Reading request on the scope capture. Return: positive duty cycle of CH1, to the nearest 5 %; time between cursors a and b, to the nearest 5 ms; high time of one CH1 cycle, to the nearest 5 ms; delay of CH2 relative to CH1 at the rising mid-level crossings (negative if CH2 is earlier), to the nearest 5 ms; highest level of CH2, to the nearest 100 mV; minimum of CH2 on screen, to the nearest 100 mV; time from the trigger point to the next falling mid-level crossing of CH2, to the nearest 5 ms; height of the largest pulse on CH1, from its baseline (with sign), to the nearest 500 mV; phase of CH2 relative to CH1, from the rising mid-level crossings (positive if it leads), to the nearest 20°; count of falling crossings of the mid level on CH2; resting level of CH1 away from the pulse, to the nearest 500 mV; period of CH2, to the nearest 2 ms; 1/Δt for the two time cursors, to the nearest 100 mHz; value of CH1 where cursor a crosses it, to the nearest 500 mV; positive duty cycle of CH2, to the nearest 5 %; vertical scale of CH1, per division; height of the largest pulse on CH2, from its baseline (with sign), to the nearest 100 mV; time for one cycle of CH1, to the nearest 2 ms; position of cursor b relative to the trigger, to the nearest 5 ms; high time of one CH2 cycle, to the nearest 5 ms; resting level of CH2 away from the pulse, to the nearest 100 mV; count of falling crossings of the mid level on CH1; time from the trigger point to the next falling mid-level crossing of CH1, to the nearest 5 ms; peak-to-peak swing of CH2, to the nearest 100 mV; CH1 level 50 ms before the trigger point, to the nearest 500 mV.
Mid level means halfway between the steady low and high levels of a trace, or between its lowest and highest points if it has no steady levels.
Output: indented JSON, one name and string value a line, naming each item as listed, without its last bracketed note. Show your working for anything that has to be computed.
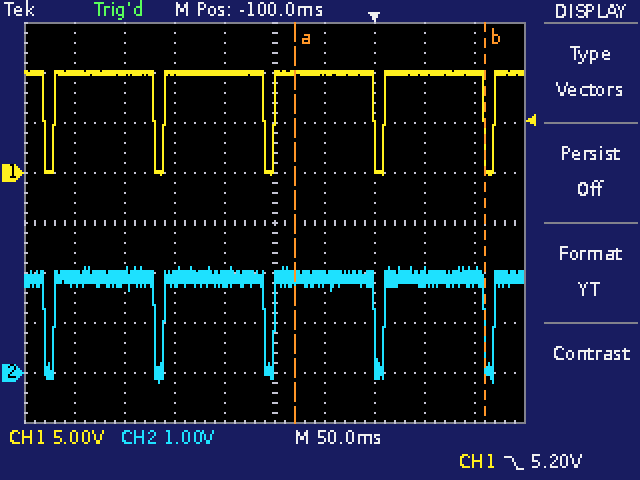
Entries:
{
  "positive duty cycle of CH1, to the nearest 5 %": "100 ms / 110 ms ≈ 90.9 %, so 90 % to the nearest 5 %",
  "time between cursors a and b, to the nearest 5 ms": "190 ms",
  "high time of one CH1 cycle, to the nearest 5 ms": "100 ms",
  "delay of CH2 relative to CH1 at the rising mid-level crossings (negative if CH2 is earlier), to the nearest 5 ms": "0 ms",
  "highest level of CH2, to the nearest 100 mV": "2.1 V",
  "minimum of CH2 on screen, to the nearest 100 mV": "-200 mV",
  "time from the trigger point to the next falling mid-level crossing of CH2, to the nearest 5 ms": "110 ms",
  "height of the largest pulse on CH1, from its baseline (with sign), to the nearest 500 mV": "-10.0 V",
  "phase of CH2 relative to CH1, from the rising mid-level crossings (positive if it leads), to the nearest 20°": "−360° × (0 ms) / 110 ms ≈ 0°",
  "count of falling crossings of the mid level on CH2": "5",
  "resting level of CH1 away from the pulse, to the nearest 500 mV": "10.0 V",
  "period of CH2, to the nearest 2 ms": "110 ms",
  "1/Δt for the two time cursors, to the nearest 100 mHz": "1 / 190 ms ≈ 5.3 Hz",
  "value of CH1 where cursor a crosses it, to the nearest 500 mV": "10.0 V",
  "positive duty cycle of CH2, to the nearest 5 %": "100 ms / 110 ms ≈ 90.9 %, so 90 % to the nearest 5 %",
  "vertical scale of CH1, per division": "5 V",
  "height of the largest pulse on CH2, from its baseline (with sign), to the nearest 100 mV": "-200 mV − (1.9 V) = -2.1 V",
  "time for one cycle of CH1, to the nearest 2 ms": "110 ms",
  "position of cursor b relative to the trigger, to the nearest 5 ms": "+110 ms",
  "high time of one CH2 cycle, to the nearest 5 ms": "100 ms",
  "resting level of CH2 away from the pulse, to the nearest 100 mV": "1.9 V",
  "count of falling crossings of the mid level on CH1": "5",
  "time from the trigger point to the next falling mid-level crossing of CH1, to the nearest 5 ms": "110 ms",
  "peak-to-peak swing of CH2, to the nearest 100 mV": "2.1 V − (-200 mV) = 2.3 V",
  "CH1 level 50 ms before the trigger point, to the nearest 500 mV": "10.0 V"
}
